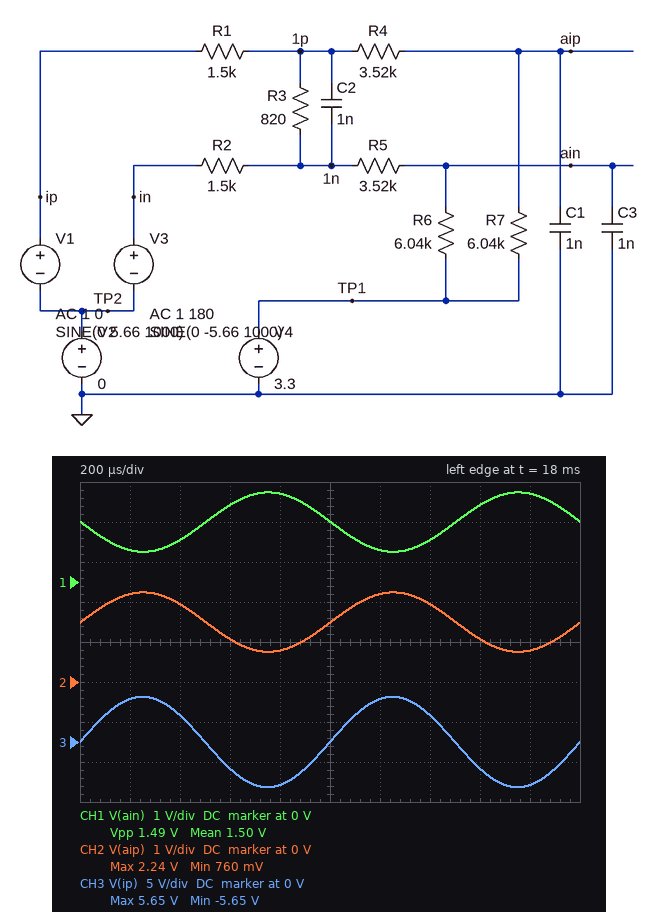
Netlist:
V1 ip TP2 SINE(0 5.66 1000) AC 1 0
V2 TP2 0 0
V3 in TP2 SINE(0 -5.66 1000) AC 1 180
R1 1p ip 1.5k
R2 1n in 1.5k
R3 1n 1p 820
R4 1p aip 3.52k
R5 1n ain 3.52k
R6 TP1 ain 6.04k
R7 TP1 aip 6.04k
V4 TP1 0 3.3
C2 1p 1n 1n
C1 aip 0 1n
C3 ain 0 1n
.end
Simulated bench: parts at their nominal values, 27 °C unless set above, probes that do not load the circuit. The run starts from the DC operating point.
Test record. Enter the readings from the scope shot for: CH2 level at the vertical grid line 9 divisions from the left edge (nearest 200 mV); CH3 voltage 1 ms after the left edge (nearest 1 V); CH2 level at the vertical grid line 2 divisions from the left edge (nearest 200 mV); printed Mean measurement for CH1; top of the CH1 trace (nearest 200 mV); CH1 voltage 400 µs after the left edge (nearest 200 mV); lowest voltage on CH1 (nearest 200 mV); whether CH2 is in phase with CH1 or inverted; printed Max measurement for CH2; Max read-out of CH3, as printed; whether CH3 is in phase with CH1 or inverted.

800 mV
0 V
2.0 V
1.50 V
2.2 V
1.0 V
800 mV
inverted
2.24 V
5.65 V
inverted
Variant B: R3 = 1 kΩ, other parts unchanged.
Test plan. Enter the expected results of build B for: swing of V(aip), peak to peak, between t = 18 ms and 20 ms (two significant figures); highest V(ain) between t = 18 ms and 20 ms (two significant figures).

1.7 V
2.4 V
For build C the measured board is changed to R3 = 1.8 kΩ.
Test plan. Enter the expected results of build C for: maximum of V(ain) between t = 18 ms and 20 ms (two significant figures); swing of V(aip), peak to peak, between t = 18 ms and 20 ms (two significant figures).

2.8 V
2.5 V
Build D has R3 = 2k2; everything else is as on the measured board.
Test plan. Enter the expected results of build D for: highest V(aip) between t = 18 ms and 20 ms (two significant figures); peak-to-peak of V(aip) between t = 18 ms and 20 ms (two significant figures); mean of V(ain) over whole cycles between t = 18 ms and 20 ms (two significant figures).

2.9 V
2.8 V
1.5 V
